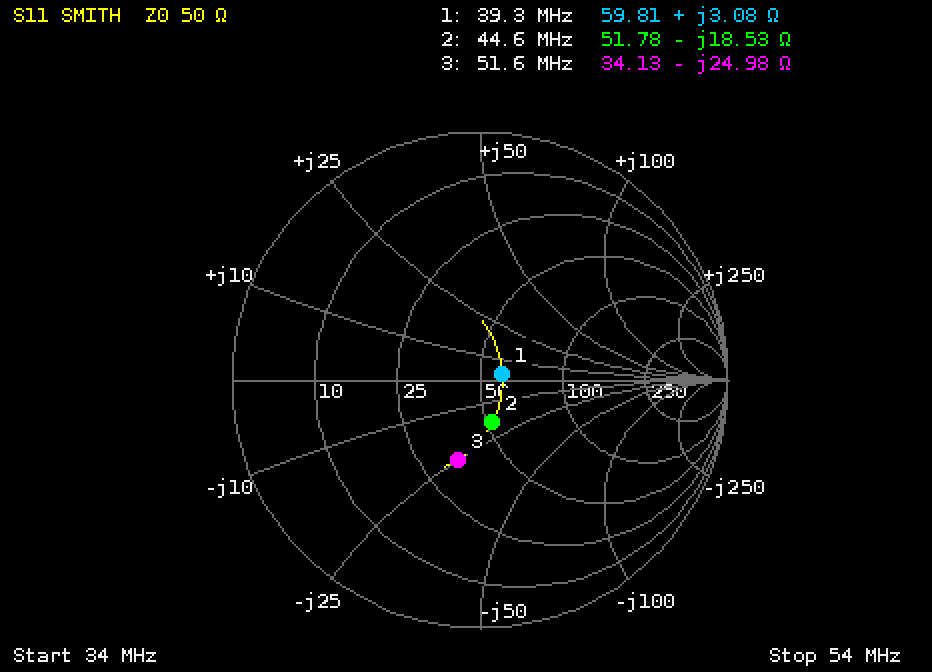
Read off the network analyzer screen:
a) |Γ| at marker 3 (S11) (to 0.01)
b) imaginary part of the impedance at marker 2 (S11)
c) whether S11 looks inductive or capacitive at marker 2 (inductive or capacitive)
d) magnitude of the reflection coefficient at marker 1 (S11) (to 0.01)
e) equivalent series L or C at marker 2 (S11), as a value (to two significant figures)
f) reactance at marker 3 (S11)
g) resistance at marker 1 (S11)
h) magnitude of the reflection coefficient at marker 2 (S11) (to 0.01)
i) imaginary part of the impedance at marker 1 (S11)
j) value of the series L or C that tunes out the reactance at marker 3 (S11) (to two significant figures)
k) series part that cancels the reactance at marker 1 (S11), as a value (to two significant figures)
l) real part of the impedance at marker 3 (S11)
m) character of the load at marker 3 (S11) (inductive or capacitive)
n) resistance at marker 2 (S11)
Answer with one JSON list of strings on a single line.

["0.34", "-18.53 Ω", "capacitive", "0.09", "190 pF", "-24.98 Ω", "59.81 Ω", "0.18", "+3.08 Ω", "77 nH", "1.3 nF", "34.13 Ω", "capacitive", "51.78 Ω"]
